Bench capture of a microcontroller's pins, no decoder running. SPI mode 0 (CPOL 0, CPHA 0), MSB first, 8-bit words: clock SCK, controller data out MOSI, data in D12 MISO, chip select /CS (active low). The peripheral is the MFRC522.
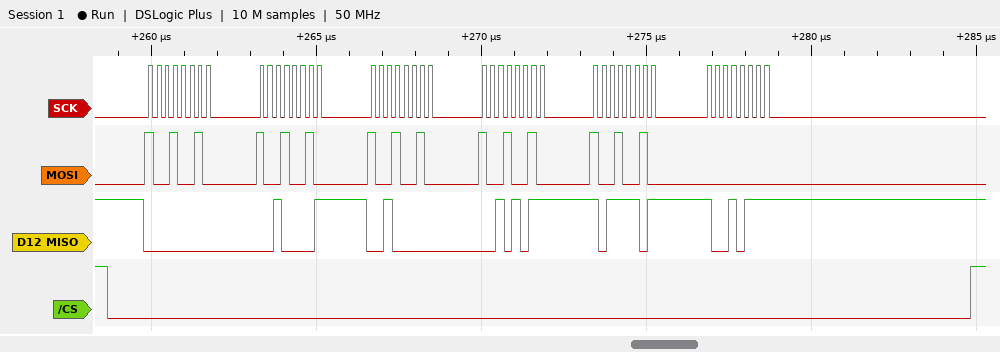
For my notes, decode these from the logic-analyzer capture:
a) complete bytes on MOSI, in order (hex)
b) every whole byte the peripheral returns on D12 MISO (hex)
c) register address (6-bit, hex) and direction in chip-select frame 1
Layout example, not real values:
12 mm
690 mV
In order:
0x92 0x92 0x92 0x92 0x92 0x00
0x00 0x21 0x20 0x2B 0xBD 0x97
0x09 read
